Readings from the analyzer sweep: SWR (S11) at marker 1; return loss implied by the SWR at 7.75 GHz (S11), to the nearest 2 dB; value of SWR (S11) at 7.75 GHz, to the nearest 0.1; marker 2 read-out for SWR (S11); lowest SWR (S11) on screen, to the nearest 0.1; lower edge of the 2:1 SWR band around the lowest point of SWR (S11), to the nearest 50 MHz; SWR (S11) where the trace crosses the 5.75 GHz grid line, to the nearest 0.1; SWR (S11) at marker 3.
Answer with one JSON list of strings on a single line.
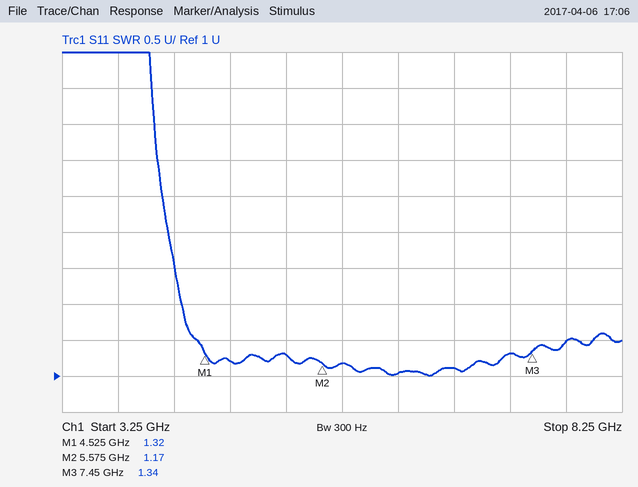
["1.32", "14 dB", "1.5", "1.17", "1.0", "4.30 GHz", "1.2", "1.34"]
